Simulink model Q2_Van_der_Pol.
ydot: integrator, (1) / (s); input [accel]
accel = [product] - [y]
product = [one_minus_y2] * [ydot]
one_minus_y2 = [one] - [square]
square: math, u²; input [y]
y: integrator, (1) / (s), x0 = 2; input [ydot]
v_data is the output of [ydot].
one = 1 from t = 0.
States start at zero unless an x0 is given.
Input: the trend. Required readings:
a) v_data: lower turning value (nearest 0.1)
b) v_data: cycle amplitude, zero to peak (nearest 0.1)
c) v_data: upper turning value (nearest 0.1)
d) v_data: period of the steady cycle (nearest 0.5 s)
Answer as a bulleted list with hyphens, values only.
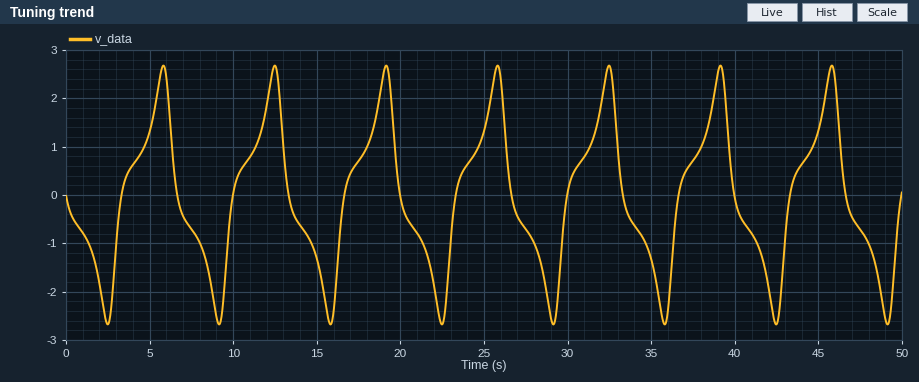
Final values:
- -2.7
- 2.7
- 2.7
- 6.5 s
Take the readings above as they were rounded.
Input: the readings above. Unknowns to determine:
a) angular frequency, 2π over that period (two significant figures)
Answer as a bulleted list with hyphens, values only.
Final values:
- 0.97 rad/s
